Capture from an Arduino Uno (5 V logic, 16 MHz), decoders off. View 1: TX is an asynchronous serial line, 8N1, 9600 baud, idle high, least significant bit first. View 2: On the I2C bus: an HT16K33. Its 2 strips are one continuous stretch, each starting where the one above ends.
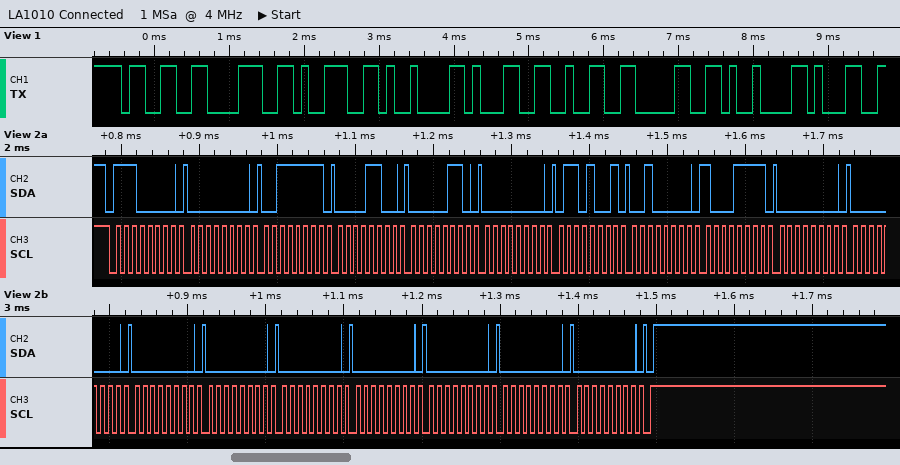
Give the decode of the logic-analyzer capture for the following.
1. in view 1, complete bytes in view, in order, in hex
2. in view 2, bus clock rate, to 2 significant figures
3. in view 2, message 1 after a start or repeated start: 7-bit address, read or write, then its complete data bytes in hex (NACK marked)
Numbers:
33 38 39 09 31 32 30 09 31
100 kHz
0x70 write: 00 3F 0C 06 00 69 20 8F 00 00 00 00 00 00 00 00 00
